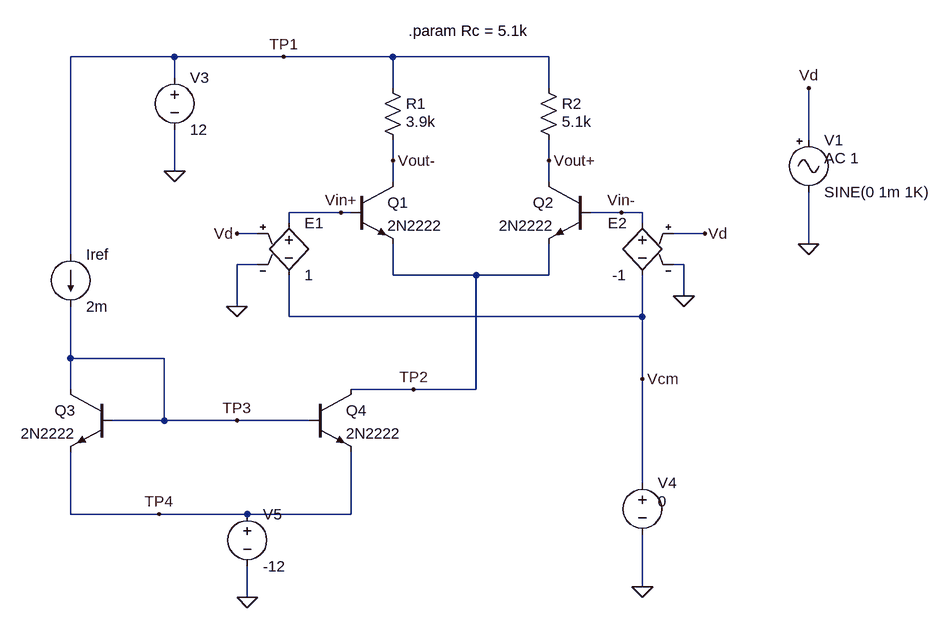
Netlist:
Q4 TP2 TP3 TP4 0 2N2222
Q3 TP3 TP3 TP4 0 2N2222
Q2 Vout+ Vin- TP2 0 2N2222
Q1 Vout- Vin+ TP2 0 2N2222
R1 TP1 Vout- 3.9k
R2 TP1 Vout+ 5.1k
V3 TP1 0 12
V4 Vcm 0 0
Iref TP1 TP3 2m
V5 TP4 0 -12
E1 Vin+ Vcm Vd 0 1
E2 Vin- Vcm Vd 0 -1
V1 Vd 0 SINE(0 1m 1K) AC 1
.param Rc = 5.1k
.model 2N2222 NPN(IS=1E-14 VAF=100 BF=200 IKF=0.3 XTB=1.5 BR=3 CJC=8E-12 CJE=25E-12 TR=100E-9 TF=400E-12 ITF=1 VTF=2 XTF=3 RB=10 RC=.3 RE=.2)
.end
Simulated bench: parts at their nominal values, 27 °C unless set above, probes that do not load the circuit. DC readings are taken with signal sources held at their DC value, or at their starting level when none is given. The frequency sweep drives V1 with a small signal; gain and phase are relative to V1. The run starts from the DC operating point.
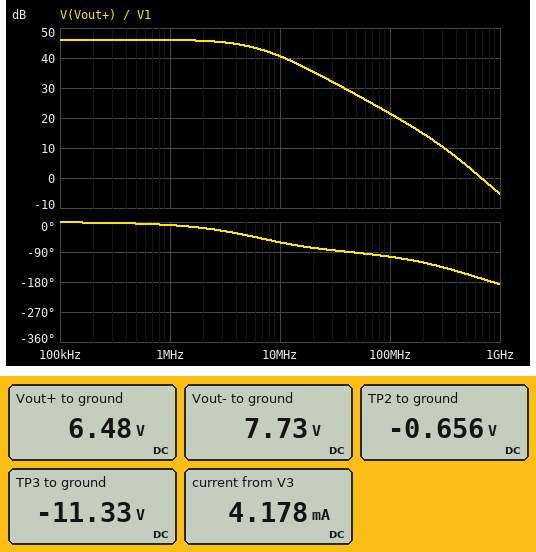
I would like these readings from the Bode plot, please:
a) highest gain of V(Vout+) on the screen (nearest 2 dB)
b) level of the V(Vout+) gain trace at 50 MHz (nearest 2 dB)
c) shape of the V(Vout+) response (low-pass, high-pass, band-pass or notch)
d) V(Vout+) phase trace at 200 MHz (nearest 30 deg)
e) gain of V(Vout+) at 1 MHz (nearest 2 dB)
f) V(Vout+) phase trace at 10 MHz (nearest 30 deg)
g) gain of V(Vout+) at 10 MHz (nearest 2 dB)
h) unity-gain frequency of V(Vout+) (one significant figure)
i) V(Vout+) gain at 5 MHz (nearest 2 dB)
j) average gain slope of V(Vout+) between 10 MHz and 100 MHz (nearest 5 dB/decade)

46 dB
28 dB
low-pass
-120 deg
46 dB
-60 deg
40 dB
700 MHz
44 dB
-20 dB/decade
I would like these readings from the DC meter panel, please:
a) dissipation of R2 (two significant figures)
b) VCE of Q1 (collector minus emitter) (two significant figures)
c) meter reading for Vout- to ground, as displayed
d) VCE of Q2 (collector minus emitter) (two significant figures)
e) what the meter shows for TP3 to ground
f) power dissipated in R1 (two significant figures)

6.0 mW
8.4 V
7.73 V
7.1 V
-11.33 V
4.7 mW
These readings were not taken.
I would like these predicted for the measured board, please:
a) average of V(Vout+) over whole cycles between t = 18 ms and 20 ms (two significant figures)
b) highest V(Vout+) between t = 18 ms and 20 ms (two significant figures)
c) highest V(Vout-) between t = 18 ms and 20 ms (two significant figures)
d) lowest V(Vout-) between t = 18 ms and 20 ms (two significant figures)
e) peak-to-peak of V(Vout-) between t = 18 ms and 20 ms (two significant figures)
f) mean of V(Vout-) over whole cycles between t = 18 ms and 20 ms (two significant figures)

6.5 V
6.7 V
7.9 V
7.6 V
310 mV
7.7 V
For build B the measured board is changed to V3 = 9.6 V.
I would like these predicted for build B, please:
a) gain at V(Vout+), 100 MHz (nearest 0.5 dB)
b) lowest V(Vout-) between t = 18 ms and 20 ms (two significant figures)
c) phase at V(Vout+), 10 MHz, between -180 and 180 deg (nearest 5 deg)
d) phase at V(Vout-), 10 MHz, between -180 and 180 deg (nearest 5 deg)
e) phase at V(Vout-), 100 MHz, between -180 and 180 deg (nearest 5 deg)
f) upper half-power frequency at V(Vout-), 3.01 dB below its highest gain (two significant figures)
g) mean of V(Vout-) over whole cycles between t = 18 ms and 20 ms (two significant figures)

20.5 dB
5.2 V
-65 deg
125 deg
75 deg
7.1 MHz
5.3 V
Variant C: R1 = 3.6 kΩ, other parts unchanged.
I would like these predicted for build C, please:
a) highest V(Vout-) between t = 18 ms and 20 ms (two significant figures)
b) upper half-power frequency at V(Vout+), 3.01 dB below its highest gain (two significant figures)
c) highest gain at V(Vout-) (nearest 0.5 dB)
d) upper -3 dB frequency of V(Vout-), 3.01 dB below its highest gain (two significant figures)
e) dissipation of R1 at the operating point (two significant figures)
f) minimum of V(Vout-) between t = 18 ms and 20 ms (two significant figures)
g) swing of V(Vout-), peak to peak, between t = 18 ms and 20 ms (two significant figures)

8.2 V
6.4 MHz
43.0 dB
8.5 MHz
4.3 mW
7.9 V
290 mV
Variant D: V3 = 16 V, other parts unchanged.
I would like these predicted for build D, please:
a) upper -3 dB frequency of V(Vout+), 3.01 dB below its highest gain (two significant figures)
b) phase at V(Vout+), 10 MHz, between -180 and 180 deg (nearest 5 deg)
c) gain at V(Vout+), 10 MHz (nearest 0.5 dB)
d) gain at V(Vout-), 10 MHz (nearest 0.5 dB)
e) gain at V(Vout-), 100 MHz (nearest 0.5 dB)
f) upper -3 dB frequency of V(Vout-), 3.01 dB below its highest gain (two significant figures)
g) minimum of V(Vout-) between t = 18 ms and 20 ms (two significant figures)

7.3 MHz
-55 deg
41.5 dB
40.5 dB
23.0 dB
9.0 MHz
12 V
